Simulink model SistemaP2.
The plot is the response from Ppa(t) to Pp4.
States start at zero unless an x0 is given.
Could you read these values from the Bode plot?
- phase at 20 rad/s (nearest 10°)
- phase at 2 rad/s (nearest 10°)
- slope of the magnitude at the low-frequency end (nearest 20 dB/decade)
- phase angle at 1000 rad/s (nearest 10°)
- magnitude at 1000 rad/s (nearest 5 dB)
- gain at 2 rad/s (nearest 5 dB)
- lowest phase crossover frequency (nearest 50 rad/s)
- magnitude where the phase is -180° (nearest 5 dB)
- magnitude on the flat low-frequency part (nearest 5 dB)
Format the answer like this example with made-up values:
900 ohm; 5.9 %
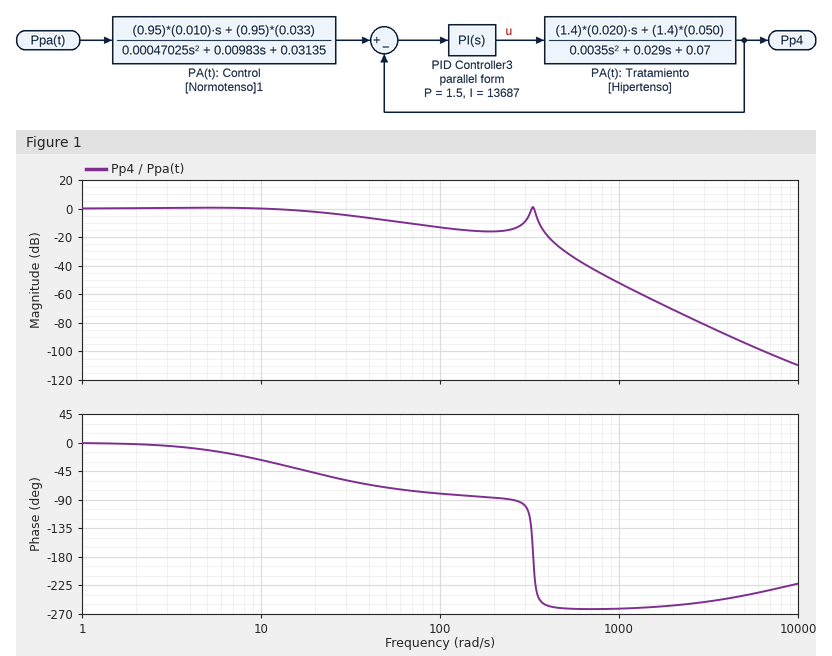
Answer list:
-50°; 0°; 0 dB/decade; -260°; -50 dB; 0 dB; 350 rad/s; 0 dB; 0 dB
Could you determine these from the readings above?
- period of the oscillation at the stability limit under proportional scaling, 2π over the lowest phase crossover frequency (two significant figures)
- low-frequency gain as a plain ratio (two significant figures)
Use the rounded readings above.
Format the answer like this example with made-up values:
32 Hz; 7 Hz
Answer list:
0.018 s; 1.0
